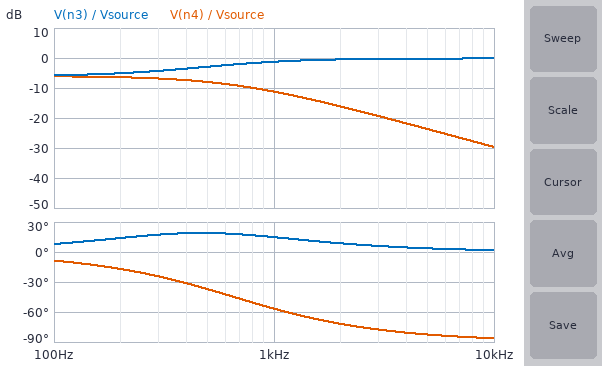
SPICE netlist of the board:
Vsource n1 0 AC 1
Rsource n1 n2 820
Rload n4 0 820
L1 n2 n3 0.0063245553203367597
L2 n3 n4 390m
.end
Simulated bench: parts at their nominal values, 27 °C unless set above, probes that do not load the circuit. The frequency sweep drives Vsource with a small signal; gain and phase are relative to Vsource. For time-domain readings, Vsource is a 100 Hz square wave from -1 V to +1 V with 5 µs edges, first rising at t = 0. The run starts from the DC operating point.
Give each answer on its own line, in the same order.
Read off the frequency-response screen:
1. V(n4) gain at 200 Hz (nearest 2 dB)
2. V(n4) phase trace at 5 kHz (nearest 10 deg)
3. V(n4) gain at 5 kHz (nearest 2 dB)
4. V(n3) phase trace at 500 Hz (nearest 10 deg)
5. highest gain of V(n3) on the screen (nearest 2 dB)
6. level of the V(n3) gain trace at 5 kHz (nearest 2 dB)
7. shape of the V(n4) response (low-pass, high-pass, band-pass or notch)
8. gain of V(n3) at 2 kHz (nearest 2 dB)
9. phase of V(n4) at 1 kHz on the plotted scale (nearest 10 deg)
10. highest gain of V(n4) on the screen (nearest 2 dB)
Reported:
-6 dB
-80 deg
-24 dB
20 deg
0 dB
0 dB
low-pass
0 dB
-60 deg
-6 dB
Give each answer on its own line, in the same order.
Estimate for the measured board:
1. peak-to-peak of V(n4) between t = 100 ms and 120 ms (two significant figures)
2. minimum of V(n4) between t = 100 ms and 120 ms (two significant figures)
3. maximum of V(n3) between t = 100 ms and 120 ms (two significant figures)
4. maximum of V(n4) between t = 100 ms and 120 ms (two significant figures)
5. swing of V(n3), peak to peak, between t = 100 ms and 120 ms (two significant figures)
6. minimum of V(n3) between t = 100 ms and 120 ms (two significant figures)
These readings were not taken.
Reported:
1.0 V
-500 mV
1.5 V
500 mV
2.9 V
-1.5 V
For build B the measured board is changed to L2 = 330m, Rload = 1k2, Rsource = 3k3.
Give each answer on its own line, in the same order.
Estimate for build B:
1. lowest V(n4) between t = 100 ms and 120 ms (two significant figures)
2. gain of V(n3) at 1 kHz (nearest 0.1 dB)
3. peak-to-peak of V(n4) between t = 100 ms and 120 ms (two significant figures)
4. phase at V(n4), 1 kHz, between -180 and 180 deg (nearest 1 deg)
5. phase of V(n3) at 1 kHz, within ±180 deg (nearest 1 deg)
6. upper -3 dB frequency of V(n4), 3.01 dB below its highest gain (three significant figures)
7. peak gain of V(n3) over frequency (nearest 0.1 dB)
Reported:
-270 mV
-6.3 dB
530 mV
-25 deg
35 deg
2.13 kHz
-0.2 dB
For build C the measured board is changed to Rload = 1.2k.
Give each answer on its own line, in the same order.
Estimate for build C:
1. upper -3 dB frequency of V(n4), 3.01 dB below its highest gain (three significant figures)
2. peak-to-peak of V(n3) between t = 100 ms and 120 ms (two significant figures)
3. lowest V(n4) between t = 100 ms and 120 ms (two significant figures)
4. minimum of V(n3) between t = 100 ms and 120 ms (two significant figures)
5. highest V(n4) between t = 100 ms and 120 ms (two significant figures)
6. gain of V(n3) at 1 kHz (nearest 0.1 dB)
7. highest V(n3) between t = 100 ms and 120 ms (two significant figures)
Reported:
811 Hz
2.7 V
-590 mV
-1.4 V
590 mV
-1.4 dB
1.4 V
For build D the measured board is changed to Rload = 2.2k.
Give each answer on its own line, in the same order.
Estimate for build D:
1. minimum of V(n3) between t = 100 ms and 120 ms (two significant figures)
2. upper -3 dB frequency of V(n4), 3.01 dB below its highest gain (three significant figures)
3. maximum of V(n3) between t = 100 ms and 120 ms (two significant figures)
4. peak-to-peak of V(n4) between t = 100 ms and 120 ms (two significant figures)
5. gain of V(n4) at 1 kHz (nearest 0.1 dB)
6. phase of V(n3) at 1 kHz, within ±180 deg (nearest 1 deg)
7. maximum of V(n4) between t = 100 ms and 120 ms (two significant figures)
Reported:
-1.2 V
1.21 kHz
1.2 V
1.5 V
-5.0 dB
9 deg
730 mV
